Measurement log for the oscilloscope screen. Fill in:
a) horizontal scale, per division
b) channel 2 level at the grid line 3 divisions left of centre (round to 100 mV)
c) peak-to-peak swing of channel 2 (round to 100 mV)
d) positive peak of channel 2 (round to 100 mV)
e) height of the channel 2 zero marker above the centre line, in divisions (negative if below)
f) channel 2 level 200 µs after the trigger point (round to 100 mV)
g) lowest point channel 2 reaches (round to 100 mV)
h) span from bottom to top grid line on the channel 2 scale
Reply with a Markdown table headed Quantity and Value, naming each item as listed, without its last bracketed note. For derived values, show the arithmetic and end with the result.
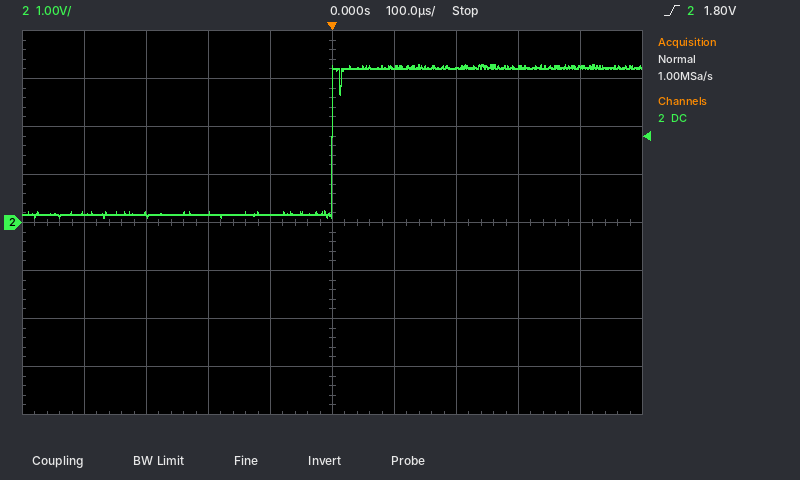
| Quantity | Value |
|---|---|
| horizontal scale, per division | 100 µs |
| channel 2 level at the grid line 3 divisions left of centre | 200 mV |
| peak-to-peak swing of channel 2 | 3.3 V − (100 mV) = 3.2 V |
| positive peak of channel 2 | 3.3 V |
| height of the channel 2 zero marker above the centre line, in divisions | 0.0 div |
| channel 2 level 200 µs after the trigger point | 3.2 V |
| lowest point channel 2 reaches | 100 mV |
| span from bottom to top grid line on the channel 2 scale | 8 V |
